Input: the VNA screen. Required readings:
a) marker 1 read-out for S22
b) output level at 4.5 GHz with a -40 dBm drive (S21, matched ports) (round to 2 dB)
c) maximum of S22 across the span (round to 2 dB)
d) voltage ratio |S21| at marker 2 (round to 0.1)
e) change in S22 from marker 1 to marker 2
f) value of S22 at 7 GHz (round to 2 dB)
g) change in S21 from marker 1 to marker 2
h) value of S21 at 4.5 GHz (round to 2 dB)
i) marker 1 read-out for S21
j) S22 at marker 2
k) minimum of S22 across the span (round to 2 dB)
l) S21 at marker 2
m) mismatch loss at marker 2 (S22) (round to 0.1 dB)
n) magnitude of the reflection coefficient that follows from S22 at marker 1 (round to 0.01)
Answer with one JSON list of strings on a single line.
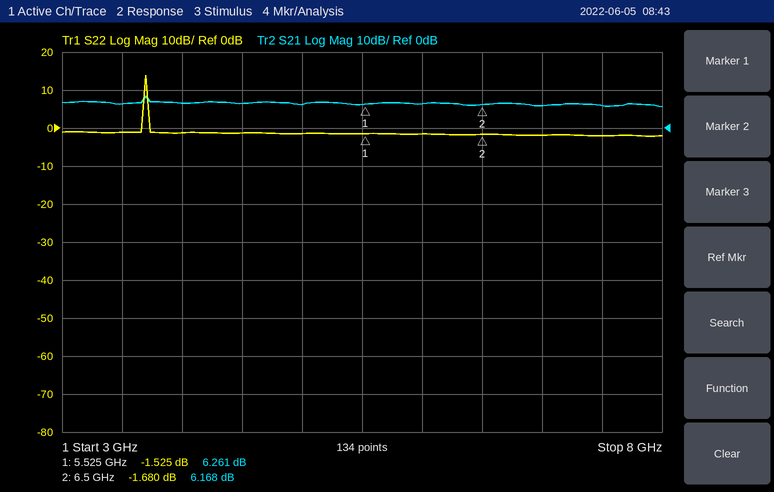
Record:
["-1.525 dB", "-34 dBm", "14 dB", "2.0", "-0.155 dB", "-2 dB", "-0.093 dB", "6 dB", "6.261 dB", "-1.680 dB", "-2 dB", "6.168 dB", "4.9 dB", "0.84"]
